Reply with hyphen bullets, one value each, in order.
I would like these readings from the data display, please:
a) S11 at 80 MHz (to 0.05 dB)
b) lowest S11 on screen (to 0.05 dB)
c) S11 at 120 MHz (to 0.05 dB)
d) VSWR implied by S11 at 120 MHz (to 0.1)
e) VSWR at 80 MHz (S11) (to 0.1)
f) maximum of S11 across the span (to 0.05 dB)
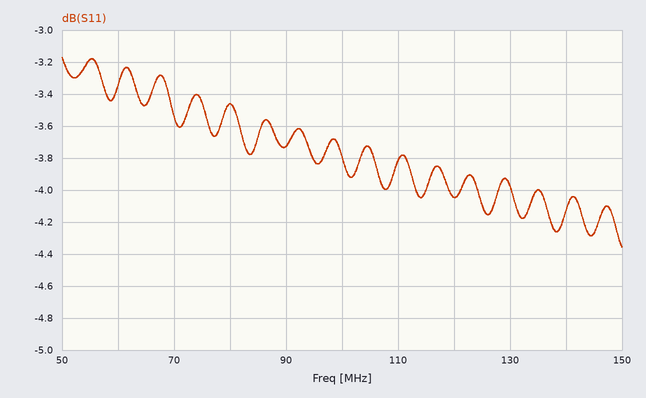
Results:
- -3.45 dB
- -4.35 dB
- -4.05 dB
- 4.4
- 5.1
- -3.15 dB
